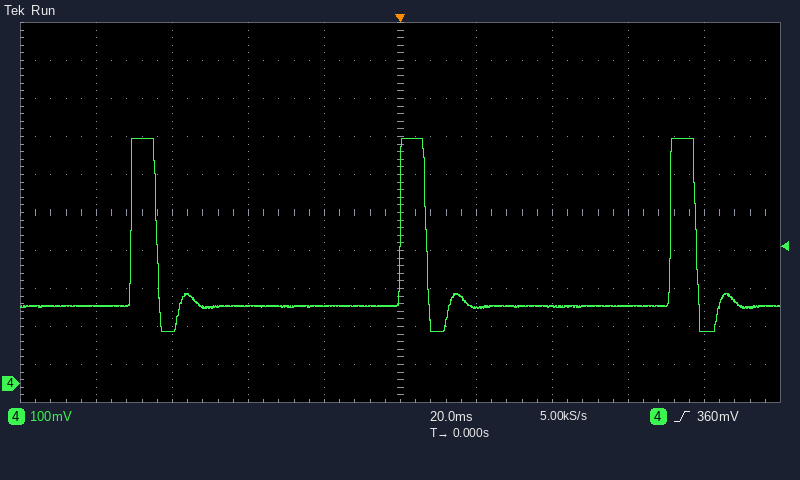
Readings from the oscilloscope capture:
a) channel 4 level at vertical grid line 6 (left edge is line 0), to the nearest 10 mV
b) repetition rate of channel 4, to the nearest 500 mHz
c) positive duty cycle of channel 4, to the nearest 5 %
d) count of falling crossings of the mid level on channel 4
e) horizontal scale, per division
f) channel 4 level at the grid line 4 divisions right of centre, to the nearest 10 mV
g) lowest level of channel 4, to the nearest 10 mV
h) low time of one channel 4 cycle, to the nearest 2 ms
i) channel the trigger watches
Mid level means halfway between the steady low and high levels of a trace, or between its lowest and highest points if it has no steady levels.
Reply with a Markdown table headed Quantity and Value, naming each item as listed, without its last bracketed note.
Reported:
| Quantity | Value |
|---|---|
| channel 4 level at vertical grid line 6 (left edge is line 0), to the nearest 10 mV | 200 mV |
| repetition rate of channel 4, to the nearest 500 mHz | 14.0 Hz |
| positive duty cycle of channel 4, to the nearest 5 % | 10 % |
| count of falling crossings of the mid level on channel 4 | 3 |
| horizontal scale, per division | 20 ms |
| channel 4 level at the grid line 4 divisions right of centre, to the nearest 10 mV | 140 mV |
| lowest level of channel 4, to the nearest 10 mV | 140 mV |
| low time of one channel 4 cycle, to the nearest 2 ms | 64 ms |
| channel the trigger watches | channel 4 |
